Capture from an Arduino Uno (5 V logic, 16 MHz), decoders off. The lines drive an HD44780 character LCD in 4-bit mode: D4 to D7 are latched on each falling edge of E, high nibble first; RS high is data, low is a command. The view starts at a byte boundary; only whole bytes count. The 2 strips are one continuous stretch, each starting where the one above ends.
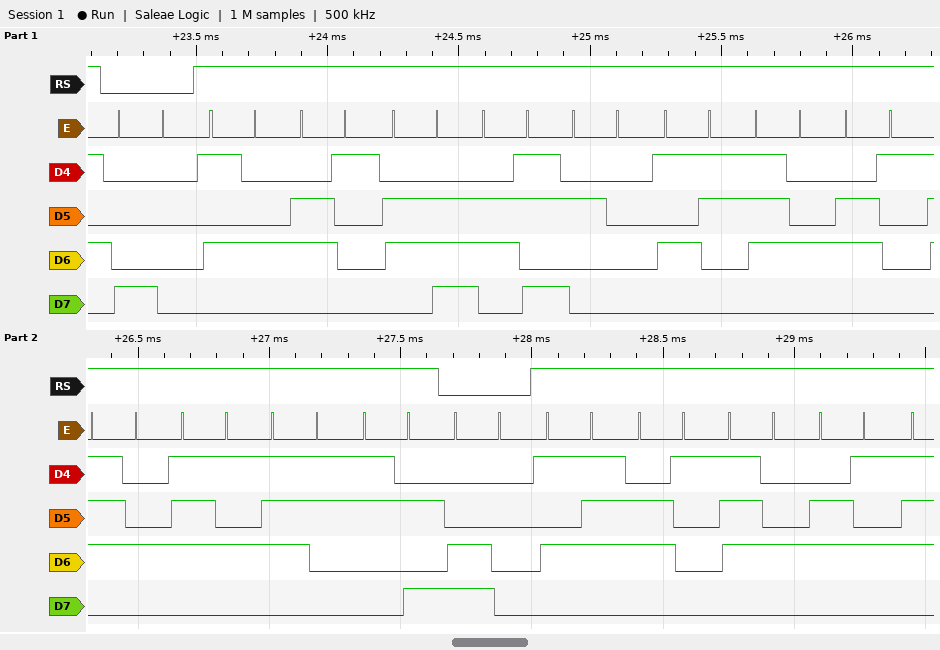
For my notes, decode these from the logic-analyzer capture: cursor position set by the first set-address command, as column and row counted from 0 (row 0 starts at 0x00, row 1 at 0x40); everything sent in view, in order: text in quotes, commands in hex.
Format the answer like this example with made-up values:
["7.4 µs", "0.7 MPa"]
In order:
["column 0, row 0", "0x80 \"Tank Status:\" 0xC0 \"Wate\""]
